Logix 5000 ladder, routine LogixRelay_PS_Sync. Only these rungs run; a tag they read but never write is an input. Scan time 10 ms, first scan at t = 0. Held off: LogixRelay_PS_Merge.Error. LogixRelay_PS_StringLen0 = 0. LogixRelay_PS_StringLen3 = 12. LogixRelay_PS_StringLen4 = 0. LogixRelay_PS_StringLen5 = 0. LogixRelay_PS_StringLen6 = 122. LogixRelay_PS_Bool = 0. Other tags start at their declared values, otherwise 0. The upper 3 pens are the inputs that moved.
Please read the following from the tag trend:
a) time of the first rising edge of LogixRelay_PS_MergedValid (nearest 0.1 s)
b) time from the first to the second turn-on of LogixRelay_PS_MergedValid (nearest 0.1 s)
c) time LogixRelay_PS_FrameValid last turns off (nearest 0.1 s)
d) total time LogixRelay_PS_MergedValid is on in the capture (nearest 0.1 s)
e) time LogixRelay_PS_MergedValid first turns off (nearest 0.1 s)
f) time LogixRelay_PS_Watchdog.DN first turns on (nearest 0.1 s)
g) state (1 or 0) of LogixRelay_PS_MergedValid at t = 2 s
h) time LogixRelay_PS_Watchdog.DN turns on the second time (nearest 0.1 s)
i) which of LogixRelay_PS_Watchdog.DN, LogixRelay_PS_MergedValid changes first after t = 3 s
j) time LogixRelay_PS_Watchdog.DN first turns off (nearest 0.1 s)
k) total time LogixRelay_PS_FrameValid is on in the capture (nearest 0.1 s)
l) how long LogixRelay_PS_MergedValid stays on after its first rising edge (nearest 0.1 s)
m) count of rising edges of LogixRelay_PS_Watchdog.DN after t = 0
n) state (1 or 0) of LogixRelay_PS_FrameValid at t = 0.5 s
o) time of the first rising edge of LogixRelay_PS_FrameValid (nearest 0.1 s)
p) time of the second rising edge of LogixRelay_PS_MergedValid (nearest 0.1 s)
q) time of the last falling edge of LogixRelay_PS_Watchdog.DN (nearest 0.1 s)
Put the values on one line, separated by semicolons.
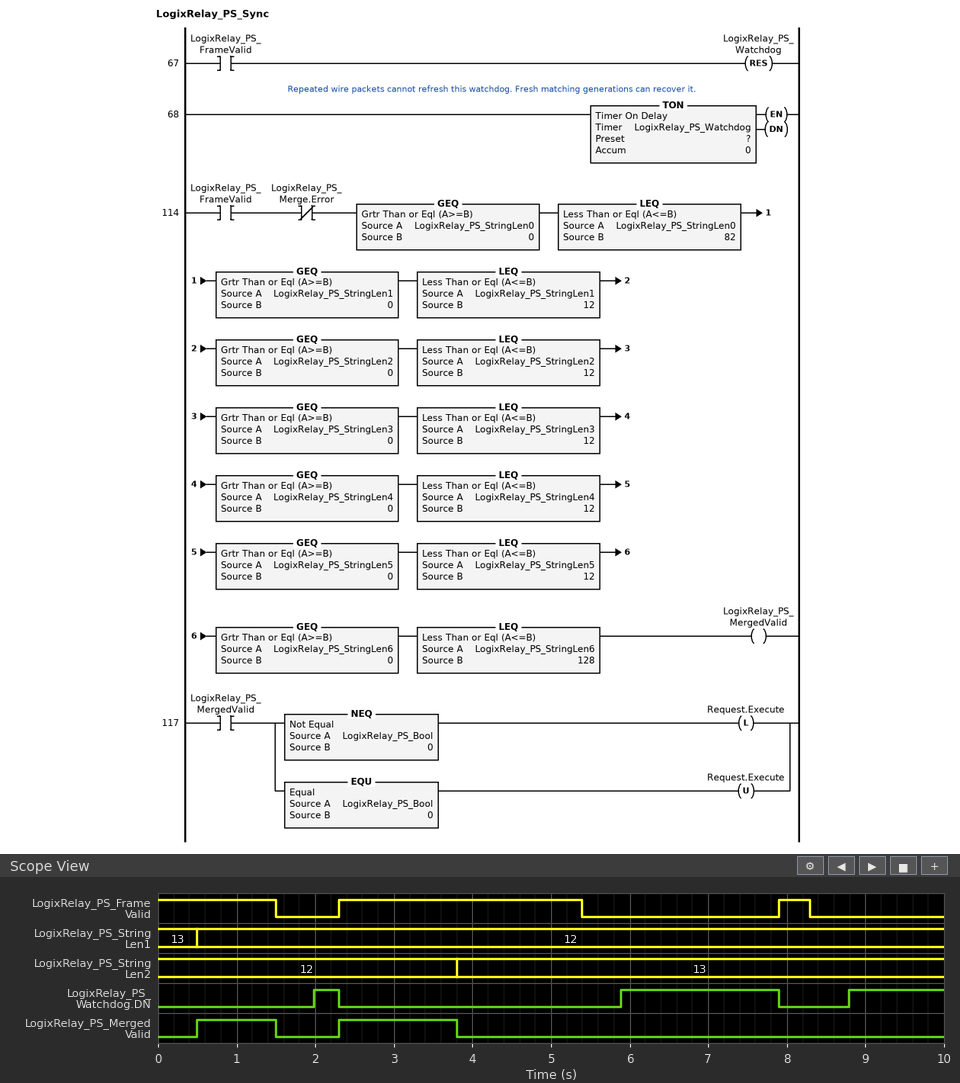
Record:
0.5 s; 1.8 s; 8.3 s; 2.5 s; 1.5 s; 2.0 s; 0; 5.9 s; LogixRelay_PS_MergedValid; 2.3 s; 5.0 s; 1.0 s; 3; 1; 2.3 s; 2.3 s; 7.9 s
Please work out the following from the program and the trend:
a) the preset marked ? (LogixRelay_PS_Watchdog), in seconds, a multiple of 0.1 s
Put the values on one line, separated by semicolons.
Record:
0.5 s
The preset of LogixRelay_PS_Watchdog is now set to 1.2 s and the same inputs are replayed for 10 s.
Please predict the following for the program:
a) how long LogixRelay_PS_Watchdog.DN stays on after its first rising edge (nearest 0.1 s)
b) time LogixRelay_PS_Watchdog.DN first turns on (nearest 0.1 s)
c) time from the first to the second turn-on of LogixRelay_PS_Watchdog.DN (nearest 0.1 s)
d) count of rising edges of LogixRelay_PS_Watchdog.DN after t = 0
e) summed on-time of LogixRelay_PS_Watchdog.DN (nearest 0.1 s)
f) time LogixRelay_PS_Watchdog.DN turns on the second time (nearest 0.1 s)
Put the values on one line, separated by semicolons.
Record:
1.3 s; 6.6 s; 2.9 s; 2; 1.8 s; 9.5 s
